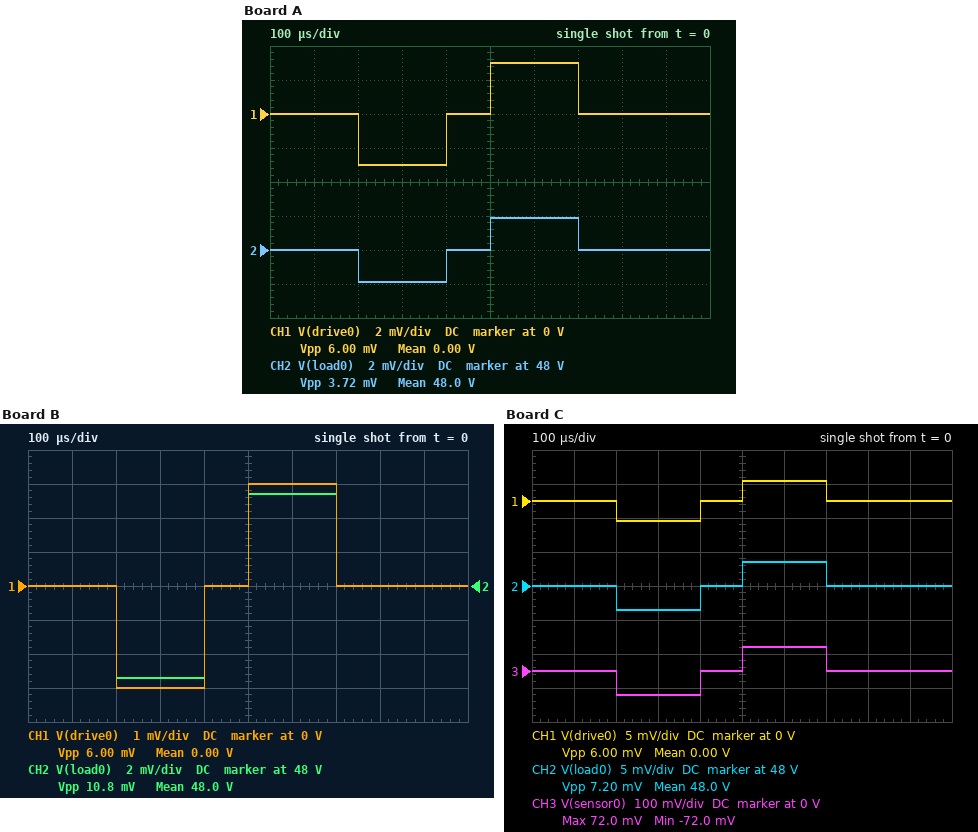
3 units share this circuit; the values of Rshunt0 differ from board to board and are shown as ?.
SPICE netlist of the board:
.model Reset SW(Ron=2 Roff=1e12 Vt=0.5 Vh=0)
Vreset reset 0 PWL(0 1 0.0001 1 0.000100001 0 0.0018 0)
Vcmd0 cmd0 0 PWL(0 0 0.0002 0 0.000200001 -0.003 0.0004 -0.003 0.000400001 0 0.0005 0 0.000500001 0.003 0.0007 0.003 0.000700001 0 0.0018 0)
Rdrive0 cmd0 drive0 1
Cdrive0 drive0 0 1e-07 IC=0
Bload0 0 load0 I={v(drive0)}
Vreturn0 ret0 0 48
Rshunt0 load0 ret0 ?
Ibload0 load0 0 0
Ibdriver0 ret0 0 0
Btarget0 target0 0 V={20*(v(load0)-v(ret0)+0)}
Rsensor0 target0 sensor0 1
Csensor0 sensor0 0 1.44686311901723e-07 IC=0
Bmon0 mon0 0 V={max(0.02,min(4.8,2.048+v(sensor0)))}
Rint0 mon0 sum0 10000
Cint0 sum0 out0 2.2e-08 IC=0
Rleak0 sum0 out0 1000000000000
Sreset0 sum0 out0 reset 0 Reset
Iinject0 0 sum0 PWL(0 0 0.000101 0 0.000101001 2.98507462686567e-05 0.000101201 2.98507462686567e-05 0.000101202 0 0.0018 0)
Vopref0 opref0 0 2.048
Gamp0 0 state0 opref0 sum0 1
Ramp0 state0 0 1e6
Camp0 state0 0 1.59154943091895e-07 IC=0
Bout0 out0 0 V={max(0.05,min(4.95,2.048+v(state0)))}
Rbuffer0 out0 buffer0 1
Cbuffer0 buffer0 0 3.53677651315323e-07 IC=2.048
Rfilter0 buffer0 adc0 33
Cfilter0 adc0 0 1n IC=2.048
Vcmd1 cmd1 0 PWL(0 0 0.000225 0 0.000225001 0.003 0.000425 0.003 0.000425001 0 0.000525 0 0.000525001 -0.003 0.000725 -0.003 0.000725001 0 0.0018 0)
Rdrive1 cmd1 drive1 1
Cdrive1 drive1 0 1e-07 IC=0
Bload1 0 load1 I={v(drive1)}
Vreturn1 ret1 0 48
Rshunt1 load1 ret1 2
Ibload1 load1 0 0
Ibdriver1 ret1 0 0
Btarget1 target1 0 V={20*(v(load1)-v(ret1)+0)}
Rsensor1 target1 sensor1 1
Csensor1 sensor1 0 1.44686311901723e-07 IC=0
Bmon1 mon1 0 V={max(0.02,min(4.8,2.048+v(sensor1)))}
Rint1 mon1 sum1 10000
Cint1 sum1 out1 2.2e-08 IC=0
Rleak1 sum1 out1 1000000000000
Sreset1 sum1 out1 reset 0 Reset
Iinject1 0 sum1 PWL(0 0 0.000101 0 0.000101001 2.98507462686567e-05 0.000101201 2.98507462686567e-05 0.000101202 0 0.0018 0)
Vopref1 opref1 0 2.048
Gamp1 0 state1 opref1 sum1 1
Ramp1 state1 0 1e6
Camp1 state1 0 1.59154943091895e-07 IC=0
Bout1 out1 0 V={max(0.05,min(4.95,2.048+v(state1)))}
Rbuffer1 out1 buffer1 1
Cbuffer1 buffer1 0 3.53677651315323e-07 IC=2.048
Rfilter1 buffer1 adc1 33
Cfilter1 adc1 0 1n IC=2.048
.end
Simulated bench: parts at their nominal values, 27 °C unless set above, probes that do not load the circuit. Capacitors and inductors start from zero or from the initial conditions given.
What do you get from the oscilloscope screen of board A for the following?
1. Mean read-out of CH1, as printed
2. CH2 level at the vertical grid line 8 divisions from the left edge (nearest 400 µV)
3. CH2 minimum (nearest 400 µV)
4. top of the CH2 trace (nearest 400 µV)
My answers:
0.00 V
48.0000 V
47.9980 V
48.0020 V
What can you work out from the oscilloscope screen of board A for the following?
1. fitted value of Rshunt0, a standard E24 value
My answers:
0.62 Ω
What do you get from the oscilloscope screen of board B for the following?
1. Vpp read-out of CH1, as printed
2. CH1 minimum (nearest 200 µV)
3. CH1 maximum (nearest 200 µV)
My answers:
6.00 mV
-3.0 mV
3.0 mV
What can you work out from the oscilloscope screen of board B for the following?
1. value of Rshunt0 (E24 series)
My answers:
1.8 Ω
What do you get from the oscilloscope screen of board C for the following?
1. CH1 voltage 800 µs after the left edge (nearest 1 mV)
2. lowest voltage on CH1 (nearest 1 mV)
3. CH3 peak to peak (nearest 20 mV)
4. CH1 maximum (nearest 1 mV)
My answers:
0 V
-3 mV
140 mV
3 mV
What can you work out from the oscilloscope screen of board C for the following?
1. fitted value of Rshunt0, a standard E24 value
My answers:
1.2 Ω
